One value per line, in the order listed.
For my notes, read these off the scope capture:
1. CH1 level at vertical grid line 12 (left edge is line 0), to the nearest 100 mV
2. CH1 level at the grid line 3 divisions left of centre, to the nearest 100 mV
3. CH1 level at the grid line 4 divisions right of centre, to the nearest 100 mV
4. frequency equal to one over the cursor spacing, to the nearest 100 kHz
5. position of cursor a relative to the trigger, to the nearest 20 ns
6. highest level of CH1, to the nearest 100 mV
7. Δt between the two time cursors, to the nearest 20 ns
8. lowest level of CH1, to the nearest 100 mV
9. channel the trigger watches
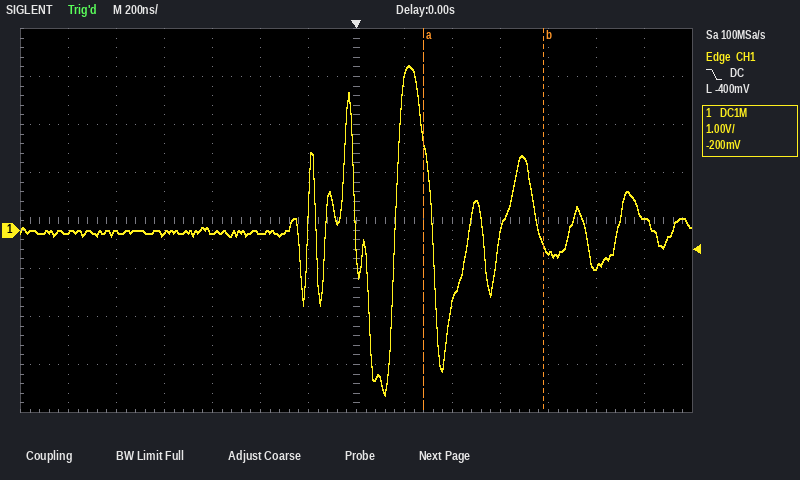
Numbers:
-800 mV
-100 mV
-500 mV
2.0 MHz
+280 ns
3.4 V
500 ns
-3.4 V
CH1
